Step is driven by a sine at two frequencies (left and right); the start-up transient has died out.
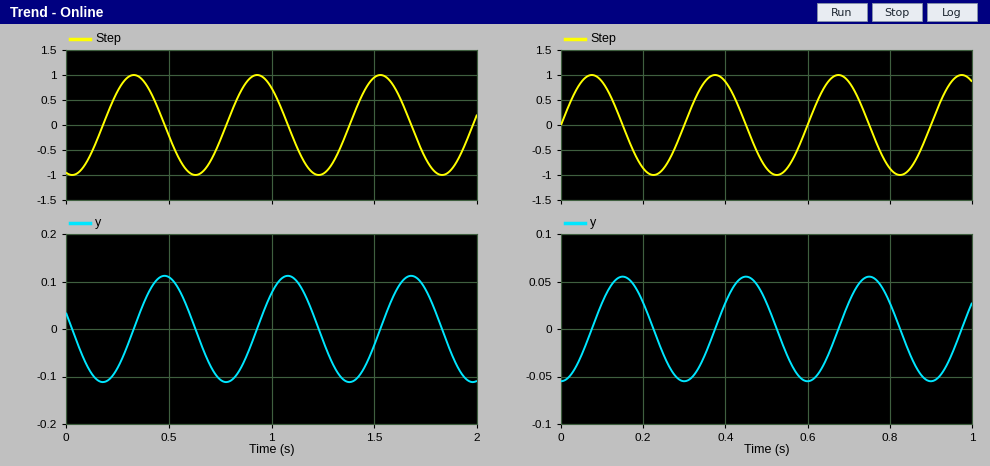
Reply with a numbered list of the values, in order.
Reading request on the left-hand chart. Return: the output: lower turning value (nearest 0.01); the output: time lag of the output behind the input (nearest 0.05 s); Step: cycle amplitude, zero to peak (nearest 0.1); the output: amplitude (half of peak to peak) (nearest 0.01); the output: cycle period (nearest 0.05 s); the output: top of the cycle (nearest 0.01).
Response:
1. -0.11
2. 0.15 s
3. 1.0
4. 0.11
5. 0.60 s
6. 0.11
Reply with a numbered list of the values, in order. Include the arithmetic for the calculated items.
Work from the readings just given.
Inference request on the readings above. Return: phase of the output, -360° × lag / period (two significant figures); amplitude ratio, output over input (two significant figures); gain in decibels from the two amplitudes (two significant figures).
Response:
1. -360 × 0.15 / 0.6 = -90°
2. 0.11 / 1 = 0.11
3. 20 log10(0.11 / 1) = -19 dB
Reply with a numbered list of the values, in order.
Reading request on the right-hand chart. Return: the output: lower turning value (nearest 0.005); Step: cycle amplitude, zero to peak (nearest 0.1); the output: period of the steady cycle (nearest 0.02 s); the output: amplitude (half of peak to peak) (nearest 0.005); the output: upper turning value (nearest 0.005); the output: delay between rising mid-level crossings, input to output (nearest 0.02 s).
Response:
1. -0.055
2. 1.0
3. 0.30 s
4. 0.055
5. 0.055
6. 0.08 s
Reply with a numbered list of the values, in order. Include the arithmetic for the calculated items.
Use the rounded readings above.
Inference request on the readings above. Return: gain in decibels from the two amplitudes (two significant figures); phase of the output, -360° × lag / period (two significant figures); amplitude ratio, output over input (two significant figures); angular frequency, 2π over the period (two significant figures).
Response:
1. 20 log10(0.055 / 1) = -25 dB
2. -360 × 0.08 / 0.3 = -96°
3. 0.055 / 1 = 0.055
4. 2π / 0.3 = 21 rad/s
